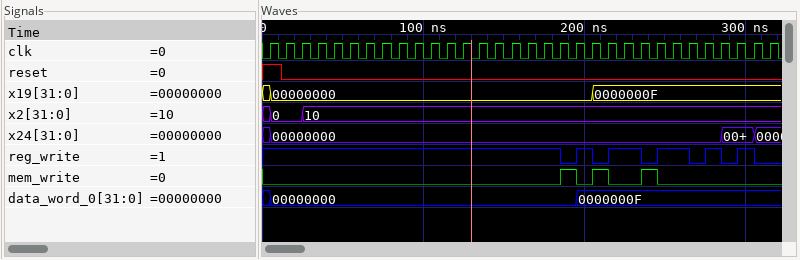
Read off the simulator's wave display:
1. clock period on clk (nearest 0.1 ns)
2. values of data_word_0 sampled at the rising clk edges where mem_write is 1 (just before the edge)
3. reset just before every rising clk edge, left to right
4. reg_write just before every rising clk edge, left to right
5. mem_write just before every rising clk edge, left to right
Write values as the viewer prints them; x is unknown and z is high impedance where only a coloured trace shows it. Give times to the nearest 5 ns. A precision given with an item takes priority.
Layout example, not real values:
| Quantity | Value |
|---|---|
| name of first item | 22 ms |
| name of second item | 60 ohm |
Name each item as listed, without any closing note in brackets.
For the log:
| Quantity | Value |
|---|---|
| clock period on clk | 10 ns |
| values of data_word_0 sampled at the rising clk edges where mem_write is 1 | 00000000, 0000000F, 0000000F |
| reset just before every rising clk edge, left to right | 1 0 0 0 0 0 0 0 0 0 0 0 0 0 0 0 0 0 0 0 0 0 0 0 0 0 0 0 0 0 0 0 |
| reg_write just before every rising clk edge, left to right | 1 1 1 1 1 1 1 1 1 1 1 1 1 1 1 1 1 1 1 0 1 0 1 1 0 1 1 0 1 0 1 0 |
| mem_write just before every rising clk edge, left to right | 0 0 0 0 0 0 0 0 0 0 0 0 0 0 0 0 0 0 0 1 0 1 0 0 1 0 0 0 0 0 0 0 |
